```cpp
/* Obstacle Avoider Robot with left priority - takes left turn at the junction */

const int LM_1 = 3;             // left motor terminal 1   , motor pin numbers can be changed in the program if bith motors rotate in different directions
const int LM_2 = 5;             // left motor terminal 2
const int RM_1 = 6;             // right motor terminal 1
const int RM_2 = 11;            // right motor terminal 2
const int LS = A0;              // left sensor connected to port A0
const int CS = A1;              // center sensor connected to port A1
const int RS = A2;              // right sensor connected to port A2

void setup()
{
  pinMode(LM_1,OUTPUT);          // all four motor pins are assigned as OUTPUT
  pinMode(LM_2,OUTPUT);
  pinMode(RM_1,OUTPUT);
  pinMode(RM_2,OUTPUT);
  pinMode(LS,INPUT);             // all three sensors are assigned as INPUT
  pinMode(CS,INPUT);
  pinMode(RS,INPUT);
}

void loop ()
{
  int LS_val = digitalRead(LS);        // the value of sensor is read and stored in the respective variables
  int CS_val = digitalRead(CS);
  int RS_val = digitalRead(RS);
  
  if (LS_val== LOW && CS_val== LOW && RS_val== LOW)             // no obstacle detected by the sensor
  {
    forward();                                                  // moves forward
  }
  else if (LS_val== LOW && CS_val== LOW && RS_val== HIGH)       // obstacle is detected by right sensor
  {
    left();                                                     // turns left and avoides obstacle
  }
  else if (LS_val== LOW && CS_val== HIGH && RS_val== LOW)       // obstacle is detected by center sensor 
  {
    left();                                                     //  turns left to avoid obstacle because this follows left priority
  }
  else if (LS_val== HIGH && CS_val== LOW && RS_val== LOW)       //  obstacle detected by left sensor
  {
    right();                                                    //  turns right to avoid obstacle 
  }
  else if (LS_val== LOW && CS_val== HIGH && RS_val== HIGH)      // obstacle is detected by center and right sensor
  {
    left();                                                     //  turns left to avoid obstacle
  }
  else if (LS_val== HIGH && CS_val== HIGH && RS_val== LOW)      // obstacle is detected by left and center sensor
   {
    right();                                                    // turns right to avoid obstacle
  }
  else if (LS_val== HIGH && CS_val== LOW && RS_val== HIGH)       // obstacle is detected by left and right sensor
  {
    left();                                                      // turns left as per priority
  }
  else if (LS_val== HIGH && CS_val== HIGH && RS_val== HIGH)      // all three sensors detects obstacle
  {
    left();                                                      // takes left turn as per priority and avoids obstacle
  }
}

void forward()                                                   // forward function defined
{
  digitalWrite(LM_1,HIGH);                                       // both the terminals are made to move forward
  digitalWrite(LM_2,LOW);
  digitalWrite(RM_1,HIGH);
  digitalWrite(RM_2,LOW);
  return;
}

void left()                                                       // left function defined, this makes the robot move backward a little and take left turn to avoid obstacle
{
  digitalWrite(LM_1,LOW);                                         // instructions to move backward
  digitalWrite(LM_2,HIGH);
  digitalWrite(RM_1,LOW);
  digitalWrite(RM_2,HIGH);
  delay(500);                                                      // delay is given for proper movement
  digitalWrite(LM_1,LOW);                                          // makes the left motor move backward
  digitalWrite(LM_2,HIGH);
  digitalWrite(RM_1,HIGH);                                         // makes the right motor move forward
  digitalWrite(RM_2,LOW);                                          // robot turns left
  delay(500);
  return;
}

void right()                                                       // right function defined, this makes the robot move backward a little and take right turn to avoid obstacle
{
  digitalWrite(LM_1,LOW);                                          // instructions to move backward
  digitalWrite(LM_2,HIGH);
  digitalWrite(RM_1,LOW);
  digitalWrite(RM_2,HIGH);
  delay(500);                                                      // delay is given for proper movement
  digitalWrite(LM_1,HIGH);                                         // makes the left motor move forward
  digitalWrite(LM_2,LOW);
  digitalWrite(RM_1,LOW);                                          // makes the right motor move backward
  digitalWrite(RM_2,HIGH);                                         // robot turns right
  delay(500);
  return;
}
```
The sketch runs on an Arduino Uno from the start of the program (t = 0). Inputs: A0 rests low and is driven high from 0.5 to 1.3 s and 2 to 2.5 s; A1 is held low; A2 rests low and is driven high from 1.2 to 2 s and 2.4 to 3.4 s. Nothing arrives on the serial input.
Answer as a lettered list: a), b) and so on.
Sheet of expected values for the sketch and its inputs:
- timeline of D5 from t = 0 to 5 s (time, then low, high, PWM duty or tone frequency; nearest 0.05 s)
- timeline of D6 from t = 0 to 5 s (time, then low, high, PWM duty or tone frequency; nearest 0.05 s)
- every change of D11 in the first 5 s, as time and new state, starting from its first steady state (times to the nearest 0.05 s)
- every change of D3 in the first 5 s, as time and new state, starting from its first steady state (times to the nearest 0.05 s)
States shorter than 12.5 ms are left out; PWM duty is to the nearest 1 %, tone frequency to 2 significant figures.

a) 0 s low; 0.5 s high; 1 s low; 1.5 s high; 3.5 s low
b) 0 s high; 0.5 s low; 2 s high; 2.5 s low; 3 s high
c) 0 s low; 0.5 s high; 2 s low; 2.5 s high; 3 s low
d) 0 s high; 0.5 s low; 1 s high; 1.5 s low; 3.5 s high
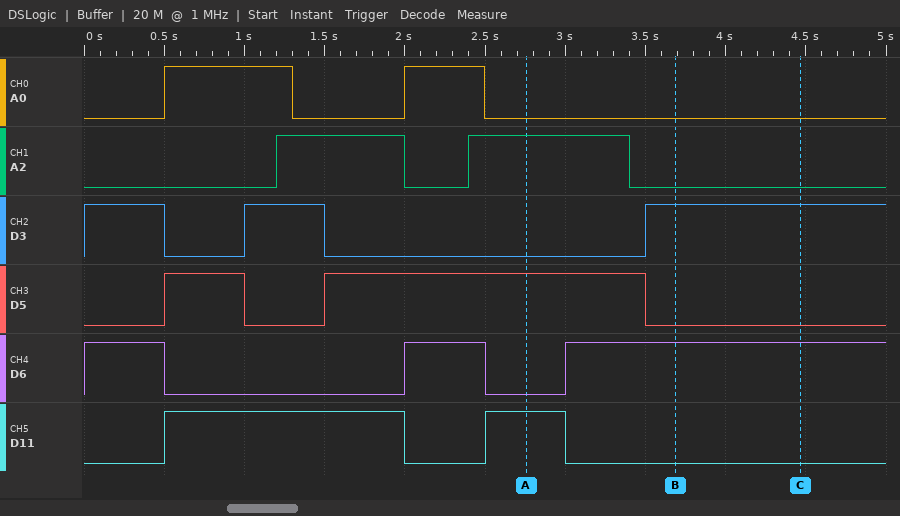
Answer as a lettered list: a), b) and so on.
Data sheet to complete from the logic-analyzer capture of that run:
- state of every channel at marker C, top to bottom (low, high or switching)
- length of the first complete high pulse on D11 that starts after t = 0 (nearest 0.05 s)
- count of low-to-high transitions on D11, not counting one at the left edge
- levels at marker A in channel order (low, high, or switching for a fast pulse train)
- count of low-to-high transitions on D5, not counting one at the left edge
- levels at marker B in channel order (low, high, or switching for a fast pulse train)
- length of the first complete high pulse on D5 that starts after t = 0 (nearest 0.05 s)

a) A0 low, A2 low, D3 high, D5 low, D6 high, D11 low
b) 1.50 s
c) 2
d) A0 low, A2 high, D3 low, D5 high, D6 low, D11 high
e) 2
f) A0 low, A2 low, D3 high, D5 low, D6 high, D11 low
g) 0.50 s
